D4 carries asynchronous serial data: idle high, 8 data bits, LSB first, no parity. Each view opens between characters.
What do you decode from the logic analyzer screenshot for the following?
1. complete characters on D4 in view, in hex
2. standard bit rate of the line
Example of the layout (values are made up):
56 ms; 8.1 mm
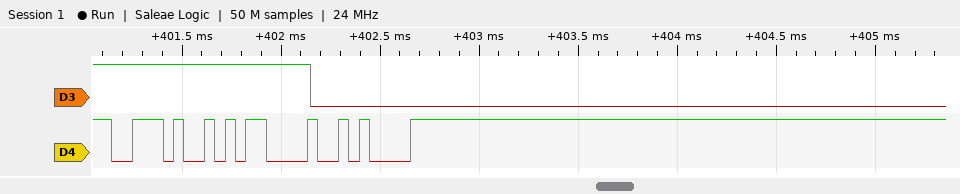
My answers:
2E, 0D, 0A; 19200 baud
